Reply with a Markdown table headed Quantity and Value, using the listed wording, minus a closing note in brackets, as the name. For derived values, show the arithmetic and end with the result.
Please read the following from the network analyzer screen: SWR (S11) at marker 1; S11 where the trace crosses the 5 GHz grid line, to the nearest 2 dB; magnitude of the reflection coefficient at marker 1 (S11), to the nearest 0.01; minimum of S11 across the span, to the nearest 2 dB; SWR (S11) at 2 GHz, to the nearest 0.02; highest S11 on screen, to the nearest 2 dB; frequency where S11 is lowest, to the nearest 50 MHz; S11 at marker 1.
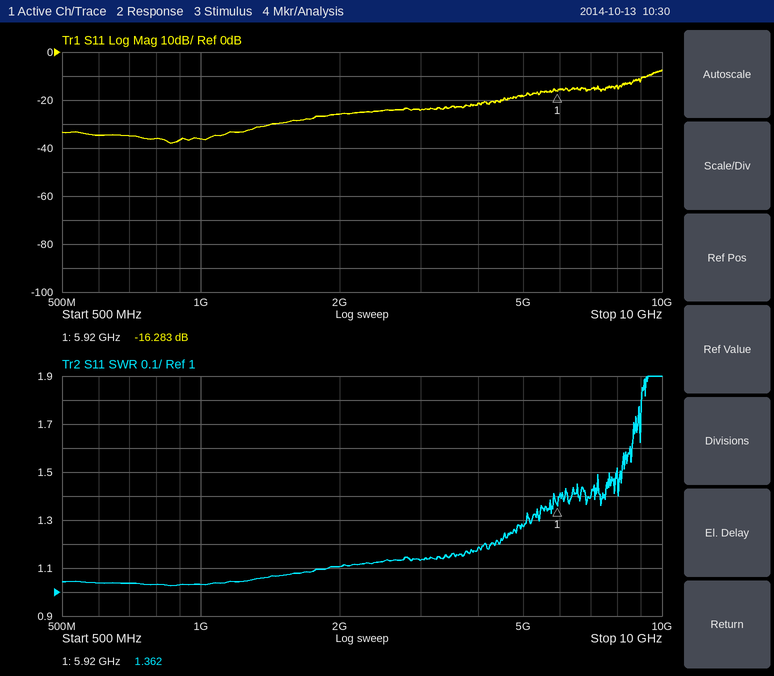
| Quantity | Value |
|---|---|
| SWR (S11) at marker 1 | 1.362 |
| S11 where the trace crosses the 5 GHz grid line, to the nearest 2 dB | -18 dB |
| magnitude of the reflection coefficient at marker 1 (S11), to the nearest 0.01 | 10^(-16.283/20) ≈ 0.15 |
| minimum of S11 across the span, to the nearest 2 dB | -38 dB |
| SWR (S11) at 2 GHz, to the nearest 0.02 | 1.10 |
| highest S11 on screen, to the nearest 2 dB | -8 dB |
| frequency where S11 is lowest, to the nearest 50 MHz | 850 MHz |
| S11 at marker 1 | -16.283 dB |
